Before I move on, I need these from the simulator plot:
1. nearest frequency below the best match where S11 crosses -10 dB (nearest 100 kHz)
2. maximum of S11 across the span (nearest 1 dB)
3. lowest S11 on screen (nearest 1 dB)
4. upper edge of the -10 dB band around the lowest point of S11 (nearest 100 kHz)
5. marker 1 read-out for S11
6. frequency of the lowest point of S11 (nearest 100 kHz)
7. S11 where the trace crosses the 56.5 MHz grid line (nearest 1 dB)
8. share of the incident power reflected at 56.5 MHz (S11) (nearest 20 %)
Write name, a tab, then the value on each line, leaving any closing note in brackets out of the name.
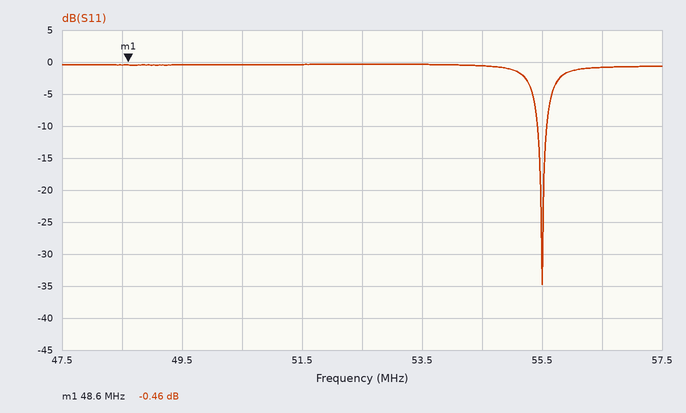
nearest frequency below the best match where S11 crosses -10 dB	55.4 MHz
maximum of S11 across the span	0 dB
lowest S11 on screen	-35 dB
upper edge of the -10 dB band around the lowest point of S11	55.6 MHz
marker 1 read-out for S11	-0.46 dB
frequency of the lowest point of S11	55.5 MHz
S11 where the trace crosses the 56.5 MHz grid line	-1 dB
share of the incident power reflected at 56.5 MHz (S11)	80 %
